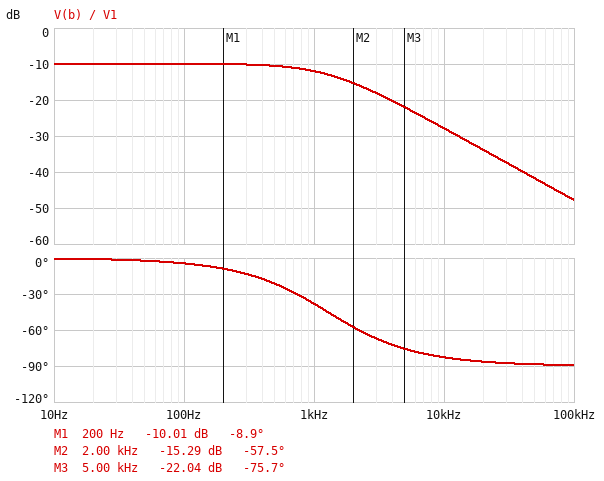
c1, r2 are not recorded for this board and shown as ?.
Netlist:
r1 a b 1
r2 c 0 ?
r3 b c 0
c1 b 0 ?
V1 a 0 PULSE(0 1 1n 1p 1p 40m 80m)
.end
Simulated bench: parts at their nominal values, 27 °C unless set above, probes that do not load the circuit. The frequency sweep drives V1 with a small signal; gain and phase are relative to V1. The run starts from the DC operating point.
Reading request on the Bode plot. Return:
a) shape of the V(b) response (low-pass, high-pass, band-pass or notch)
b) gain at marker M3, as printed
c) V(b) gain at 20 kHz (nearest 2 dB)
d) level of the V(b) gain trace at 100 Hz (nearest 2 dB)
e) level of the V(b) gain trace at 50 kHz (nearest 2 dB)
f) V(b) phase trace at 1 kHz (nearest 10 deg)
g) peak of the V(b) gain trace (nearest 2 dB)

low-pass
-22.04 dB
-34 dB
-10 dB
-42 dB
-40 deg
-10 dB
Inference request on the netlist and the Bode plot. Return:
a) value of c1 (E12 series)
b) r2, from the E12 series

390 µF
0.47 Ω
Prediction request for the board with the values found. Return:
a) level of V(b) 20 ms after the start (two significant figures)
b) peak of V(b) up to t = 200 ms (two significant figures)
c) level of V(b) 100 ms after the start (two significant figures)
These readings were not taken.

320 mV
320 mV
320 mV
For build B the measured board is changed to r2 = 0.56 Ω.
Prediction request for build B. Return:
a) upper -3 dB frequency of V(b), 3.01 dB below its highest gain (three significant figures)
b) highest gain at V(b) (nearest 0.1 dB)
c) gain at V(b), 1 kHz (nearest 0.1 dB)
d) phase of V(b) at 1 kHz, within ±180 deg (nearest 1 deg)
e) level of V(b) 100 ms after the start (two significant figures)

1.14 kHz
-8.9 dB
-11.4 dB
-41 deg
360 mV
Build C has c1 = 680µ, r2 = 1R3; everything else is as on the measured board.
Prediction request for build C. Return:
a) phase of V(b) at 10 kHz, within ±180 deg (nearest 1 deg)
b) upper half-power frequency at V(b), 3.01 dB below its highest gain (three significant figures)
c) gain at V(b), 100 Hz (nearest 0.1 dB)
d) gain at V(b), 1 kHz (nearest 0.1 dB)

-88 deg
414 Hz
-5.2 dB
-13.3 dB
